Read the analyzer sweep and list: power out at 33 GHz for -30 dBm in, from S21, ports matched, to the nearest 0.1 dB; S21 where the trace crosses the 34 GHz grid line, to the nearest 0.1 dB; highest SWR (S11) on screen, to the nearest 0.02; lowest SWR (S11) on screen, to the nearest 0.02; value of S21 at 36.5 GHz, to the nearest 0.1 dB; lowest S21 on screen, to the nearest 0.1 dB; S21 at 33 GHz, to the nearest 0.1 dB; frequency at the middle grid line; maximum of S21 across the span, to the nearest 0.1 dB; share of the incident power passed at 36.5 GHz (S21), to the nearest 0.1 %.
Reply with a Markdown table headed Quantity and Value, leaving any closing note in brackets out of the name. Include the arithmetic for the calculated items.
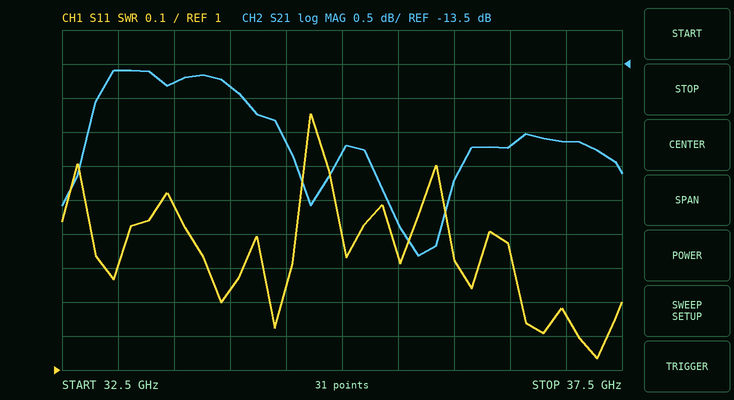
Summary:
| Quantity | Value |
|---|---|
| power out at 33 GHz for -30 dBm in, from S21, ports matched, to the nearest 0.1 dB | -30 dBm + (-13.6 dB) = -43.6 dBm |
| S21 where the trace crosses the 34 GHz grid line, to the nearest 0.1 dB | -13.8 dB |
| highest SWR (S11) on screen, to the nearest 0.02 | 1.76 |
| lowest SWR (S11) on screen, to the nearest 0.02 | 1.04 |
| value of S21 at 36.5 GHz, to the nearest 0.1 dB | -14.7 dB |
| lowest S21 on screen, to the nearest 0.1 dB | -16.3 dB |
| S21 at 33 GHz, to the nearest 0.1 dB | -13.6 dB |
| frequency at the middle grid line | 35 GHz |
| maximum of S21 across the span, to the nearest 0.1 dB | -13.6 dB |
| share of the incident power passed at 36.5 GHz (S21), to the nearest 0.1 % | 10^(-14.7/10) ≈ 3.4 % |
